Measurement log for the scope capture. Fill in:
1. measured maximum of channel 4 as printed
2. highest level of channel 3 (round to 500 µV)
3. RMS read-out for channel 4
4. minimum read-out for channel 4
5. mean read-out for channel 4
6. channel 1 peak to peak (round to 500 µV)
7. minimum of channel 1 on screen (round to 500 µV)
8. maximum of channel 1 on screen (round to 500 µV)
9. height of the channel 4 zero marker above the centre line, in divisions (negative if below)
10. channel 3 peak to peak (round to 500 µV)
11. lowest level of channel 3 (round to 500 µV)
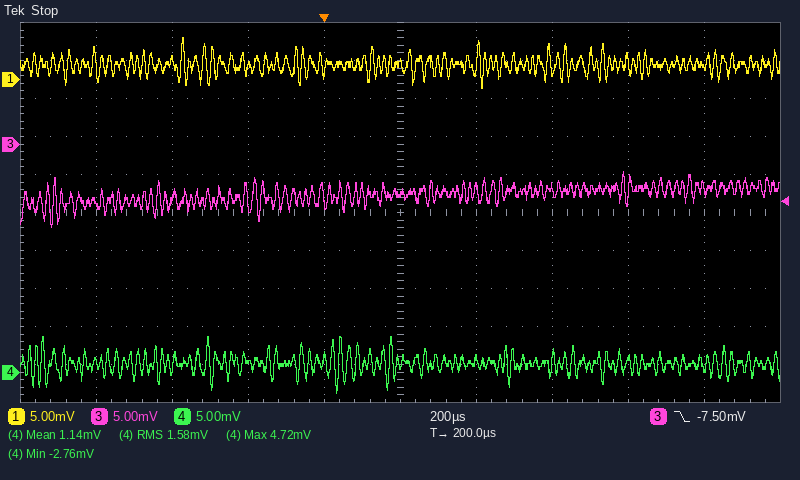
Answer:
4.72 mV
-3.5 mV
1.58 mV
-2.76 mV
1.14 mV
6.5 mV
-1.0 mV
5.5 mV
-4.2 div
7.5 mV
-11.0 mV
